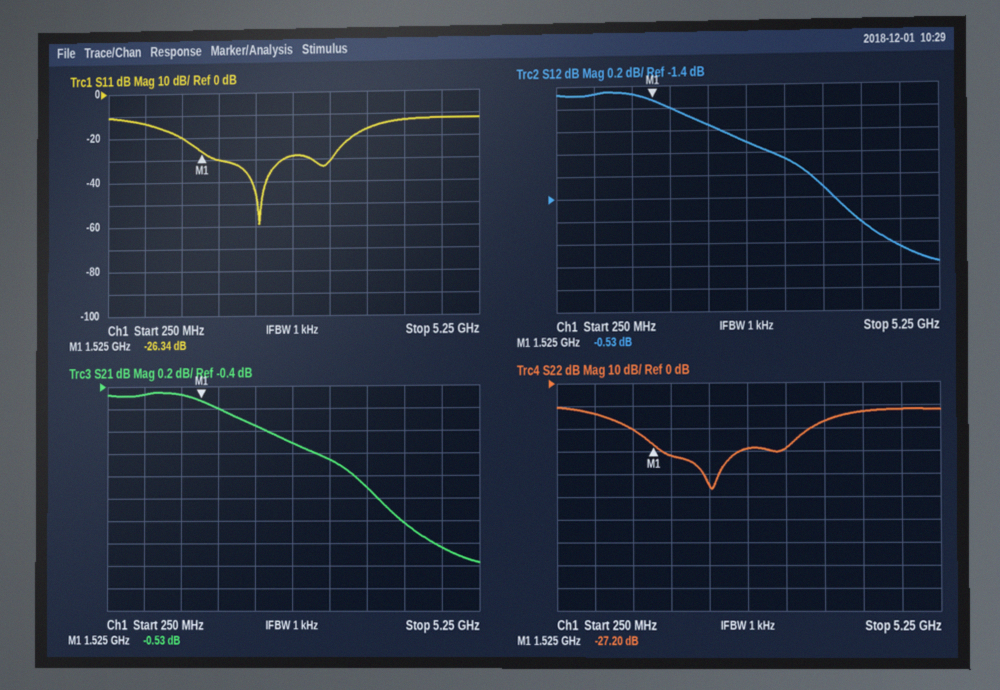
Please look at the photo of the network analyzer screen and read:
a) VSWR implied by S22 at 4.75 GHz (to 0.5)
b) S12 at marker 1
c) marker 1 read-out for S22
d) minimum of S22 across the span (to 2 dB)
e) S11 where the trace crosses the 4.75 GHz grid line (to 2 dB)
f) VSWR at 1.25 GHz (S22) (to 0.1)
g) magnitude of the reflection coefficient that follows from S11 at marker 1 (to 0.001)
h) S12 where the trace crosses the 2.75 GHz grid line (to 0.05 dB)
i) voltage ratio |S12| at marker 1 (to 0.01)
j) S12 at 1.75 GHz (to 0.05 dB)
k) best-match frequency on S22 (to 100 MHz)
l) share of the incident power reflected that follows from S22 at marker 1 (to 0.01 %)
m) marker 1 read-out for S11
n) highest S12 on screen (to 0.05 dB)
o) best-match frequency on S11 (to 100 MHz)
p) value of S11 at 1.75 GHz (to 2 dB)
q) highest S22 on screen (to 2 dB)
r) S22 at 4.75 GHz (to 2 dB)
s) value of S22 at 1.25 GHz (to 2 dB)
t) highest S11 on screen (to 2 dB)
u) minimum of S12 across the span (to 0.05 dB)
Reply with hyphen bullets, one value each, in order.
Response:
- 1.5
- -0.53 dB
- -27.20 dB
- -46 dB
- -12 dB
- 1.2
- 0.048
- -0.90 dB
- 0.94
- -0.60 dB
- 2.3 GHz
- 0.19 %
- -26.34 dB
- -0.45 dB
- 2.3 GHz
- -30 dB
- -10 dB
- -12 dB
- -20 dB
- -10 dB
- -1.95 dB
